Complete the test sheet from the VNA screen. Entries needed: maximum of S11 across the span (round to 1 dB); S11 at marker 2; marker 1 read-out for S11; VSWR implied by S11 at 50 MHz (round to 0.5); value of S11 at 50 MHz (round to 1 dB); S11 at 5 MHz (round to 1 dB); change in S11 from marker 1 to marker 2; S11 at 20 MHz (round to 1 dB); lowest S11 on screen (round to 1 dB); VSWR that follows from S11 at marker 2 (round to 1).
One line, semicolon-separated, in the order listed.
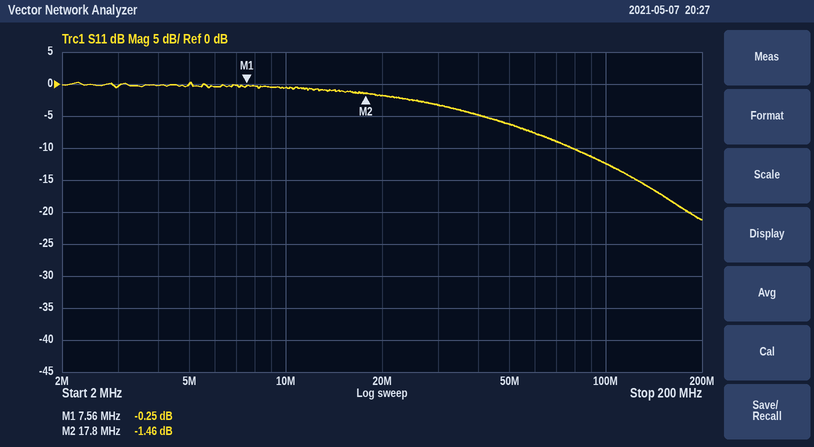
0 dB; -1.46 dB; -0.25 dB; 3.0; -6 dB; 0 dB; -1.21 dB; -2 dB; -21 dB; 12
